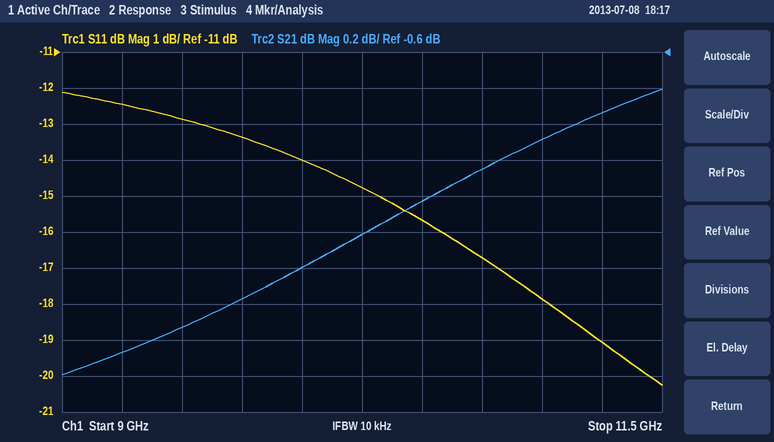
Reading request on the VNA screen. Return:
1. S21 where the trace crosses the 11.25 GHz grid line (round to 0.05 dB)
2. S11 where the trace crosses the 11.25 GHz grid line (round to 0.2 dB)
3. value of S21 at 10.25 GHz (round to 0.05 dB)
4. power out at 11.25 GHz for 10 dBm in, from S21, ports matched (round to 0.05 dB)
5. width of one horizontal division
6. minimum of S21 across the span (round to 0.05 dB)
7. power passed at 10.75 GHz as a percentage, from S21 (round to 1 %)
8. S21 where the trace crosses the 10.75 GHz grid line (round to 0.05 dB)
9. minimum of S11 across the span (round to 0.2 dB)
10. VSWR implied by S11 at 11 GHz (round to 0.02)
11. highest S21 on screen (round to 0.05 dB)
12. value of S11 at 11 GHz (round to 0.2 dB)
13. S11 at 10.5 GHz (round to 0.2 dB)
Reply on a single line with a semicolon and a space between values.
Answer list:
-0.95 dB; -19.0 dB; -1.60 dB; 9.05 dBm; 250 MHz; -2.40 dB; 75 %; -1.25 dB; -20.2 dB; 1.30; -0.80 dB; -17.8 dB; -15.6 dB
